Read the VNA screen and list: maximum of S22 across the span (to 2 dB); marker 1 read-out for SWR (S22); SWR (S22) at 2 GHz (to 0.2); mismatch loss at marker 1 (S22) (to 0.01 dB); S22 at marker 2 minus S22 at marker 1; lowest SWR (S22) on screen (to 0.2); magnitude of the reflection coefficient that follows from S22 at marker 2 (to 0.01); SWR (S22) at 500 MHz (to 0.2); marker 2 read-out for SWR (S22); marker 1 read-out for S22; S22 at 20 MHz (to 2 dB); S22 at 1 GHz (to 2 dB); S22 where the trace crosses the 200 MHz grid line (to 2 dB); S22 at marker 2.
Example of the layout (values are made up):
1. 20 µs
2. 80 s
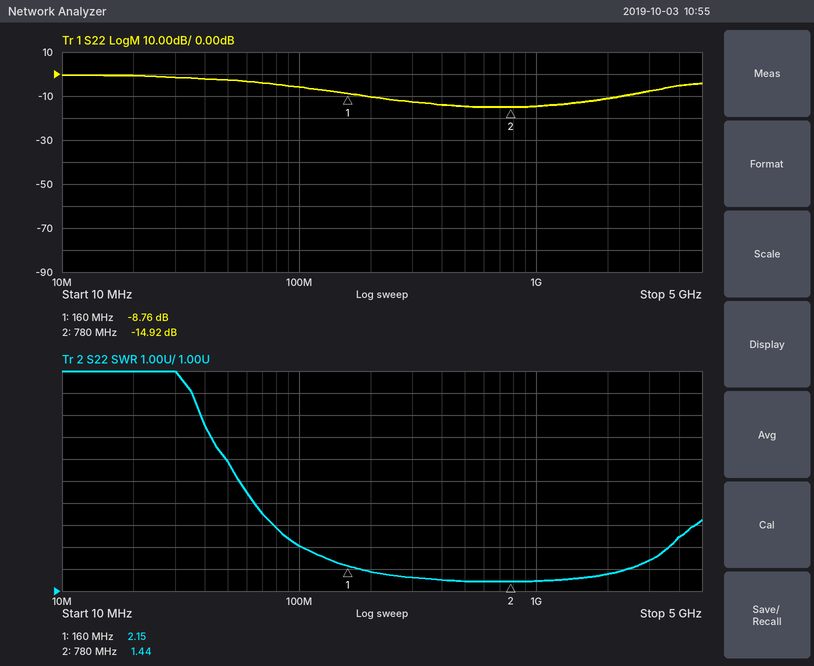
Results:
1. 0 dB
2. 2.15
3. 1.8
4. 0.62 dB
5. -6.16 dB
6. 1.4
7. 0.18
8. 1.4
9. 1.44
10. -8.76 dB
11. 0 dB
12. -14 dB
13. -10 dB
14. -14.92 dB
